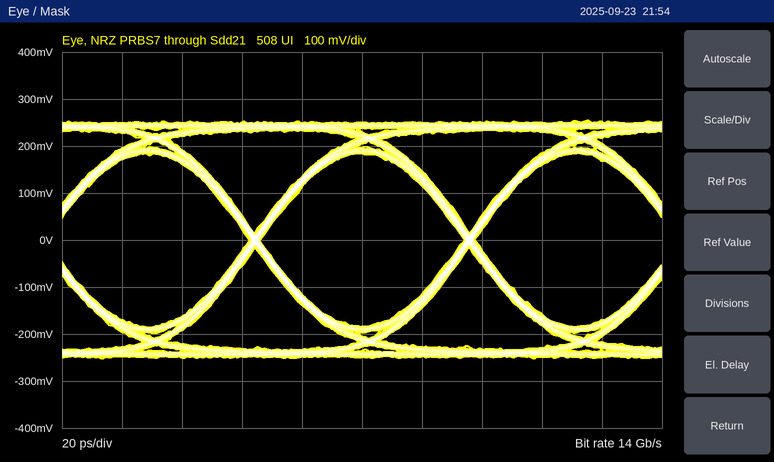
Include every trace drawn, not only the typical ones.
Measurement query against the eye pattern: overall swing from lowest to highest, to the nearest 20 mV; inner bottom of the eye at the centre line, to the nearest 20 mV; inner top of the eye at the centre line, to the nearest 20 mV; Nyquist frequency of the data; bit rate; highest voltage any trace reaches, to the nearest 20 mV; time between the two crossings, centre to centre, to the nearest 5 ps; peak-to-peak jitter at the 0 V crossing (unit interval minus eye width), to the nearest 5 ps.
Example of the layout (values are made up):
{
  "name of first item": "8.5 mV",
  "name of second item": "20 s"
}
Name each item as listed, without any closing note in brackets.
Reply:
{
  "overall swing from lowest to highest, to the nearest 20 mV": "500 mV",
  "inner bottom of the eye at the centre line, to the nearest 20 mV": "-180 mV",
  "inner top of the eye at the centre line, to the nearest 20 mV": "180 mV",
  "Nyquist frequency of the data": "7 GHz",
  "bit rate": "14 Gb/s",
  "highest voltage any trace reaches, to the nearest 20 mV": "260 mV",
  "time between the two crossings, centre to centre, to the nearest 5 ps": "70 ps",
  "peak-to-peak jitter at the 0 V crossing (unit interval minus eye width), to the nearest 5 ps": "5 ps"
}
